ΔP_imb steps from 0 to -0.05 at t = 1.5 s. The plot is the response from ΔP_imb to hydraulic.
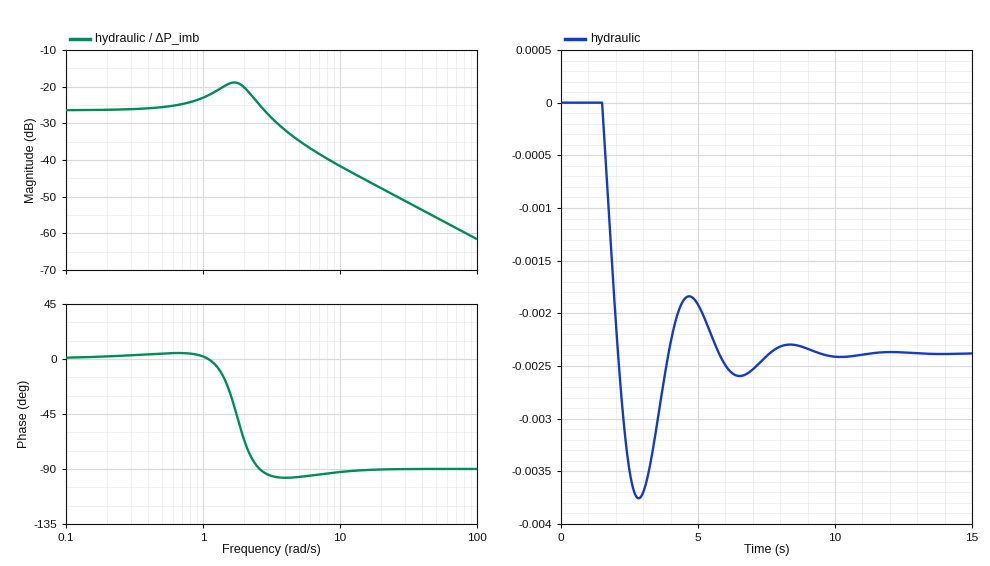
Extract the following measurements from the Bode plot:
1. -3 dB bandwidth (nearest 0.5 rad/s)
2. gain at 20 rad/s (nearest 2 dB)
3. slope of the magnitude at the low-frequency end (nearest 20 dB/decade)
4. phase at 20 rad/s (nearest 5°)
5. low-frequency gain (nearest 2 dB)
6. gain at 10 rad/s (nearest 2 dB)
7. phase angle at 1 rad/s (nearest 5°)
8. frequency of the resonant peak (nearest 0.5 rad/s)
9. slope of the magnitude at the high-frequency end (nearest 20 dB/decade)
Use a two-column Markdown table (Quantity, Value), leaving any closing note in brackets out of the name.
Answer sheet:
| Quantity | Value |
|---|---|
| -3 dB bandwidth | 3.5 rad/s |
| gain at 20 rad/s | -48 dB |
| slope of the magnitude at the low-frequency end | 0 dB/decade |
| phase at 20 rad/s | -90° |
| low-frequency gain | -26 dB |
| gain at 10 rad/s | -42 dB |
| phase angle at 1 rad/s | 0° |
| frequency of the resonant peak | 1.5 rad/s |
| slope of the magnitude at the high-frequency end | -20 dB/decade |
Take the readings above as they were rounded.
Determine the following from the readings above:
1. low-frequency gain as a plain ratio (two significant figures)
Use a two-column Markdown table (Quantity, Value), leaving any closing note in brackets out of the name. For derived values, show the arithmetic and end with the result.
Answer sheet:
| Quantity | Value |
|---|---|
| low-frequency gain as a plain ratio | 10^(-26 / 20) = 0.050 |
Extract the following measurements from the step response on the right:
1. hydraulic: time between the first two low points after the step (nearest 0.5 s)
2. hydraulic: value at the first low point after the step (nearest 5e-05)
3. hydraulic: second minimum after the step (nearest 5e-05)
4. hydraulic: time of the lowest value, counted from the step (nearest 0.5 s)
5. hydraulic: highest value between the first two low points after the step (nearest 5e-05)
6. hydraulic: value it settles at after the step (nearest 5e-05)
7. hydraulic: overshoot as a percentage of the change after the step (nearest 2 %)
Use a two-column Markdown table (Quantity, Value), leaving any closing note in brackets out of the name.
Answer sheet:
| Quantity | Value |
|---|---|
| hydraulic: time between the first two low points after the step | 3.5 s |
| hydraulic: value at the first low point after the step | -0.00375 |
| hydraulic: second minimum after the step | -0.00260 |
| hydraulic: time of the lowest value, counted from the step | 1.5 s |
| hydraulic: highest value between the first two low points after the step | -0.00185 |
| hydraulic: value it settles at after the step | -0.00240 |
| hydraulic: overshoot as a percentage of the change after the step | 58 % |
